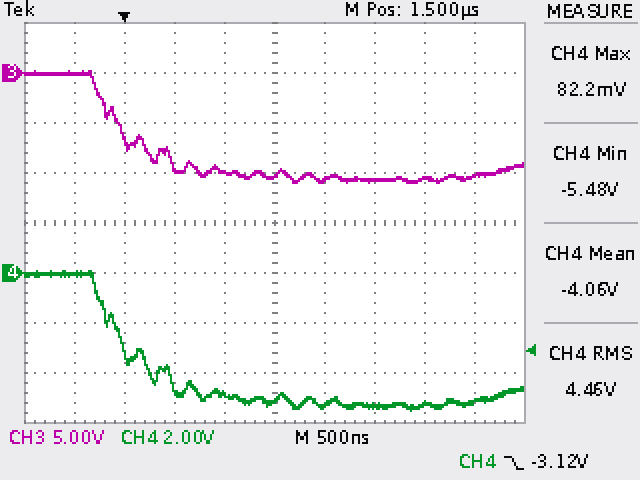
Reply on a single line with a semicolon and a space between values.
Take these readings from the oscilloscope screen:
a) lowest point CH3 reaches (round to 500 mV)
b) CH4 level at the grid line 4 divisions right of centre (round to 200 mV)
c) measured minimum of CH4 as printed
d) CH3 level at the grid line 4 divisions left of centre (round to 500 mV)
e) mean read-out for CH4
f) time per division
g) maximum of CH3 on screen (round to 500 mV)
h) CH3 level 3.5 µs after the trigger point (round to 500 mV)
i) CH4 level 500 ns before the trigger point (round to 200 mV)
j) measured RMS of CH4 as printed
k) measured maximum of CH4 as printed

-11.0 V; -5.2 V; -5.48 V; 0.0 V; -4.06 V; 500 ns; 0.0 V; -10.5 V; 0.0 V; 4.46 V; 82.2 mV
